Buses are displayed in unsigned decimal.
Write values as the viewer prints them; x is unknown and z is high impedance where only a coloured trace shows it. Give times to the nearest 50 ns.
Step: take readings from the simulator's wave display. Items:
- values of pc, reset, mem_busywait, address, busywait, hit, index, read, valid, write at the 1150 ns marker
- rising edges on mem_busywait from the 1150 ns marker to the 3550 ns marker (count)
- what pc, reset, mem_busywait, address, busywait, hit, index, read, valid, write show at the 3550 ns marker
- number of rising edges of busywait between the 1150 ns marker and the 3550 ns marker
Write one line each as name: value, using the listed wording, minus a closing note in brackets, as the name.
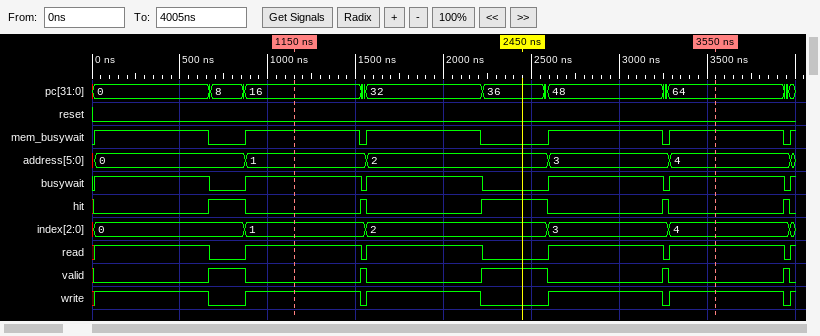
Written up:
values of pc, reset, mem_busywait, address, busywait, hit, index, read, valid, write at the 1150 ns marker: pc=16, reset=0, mem_busywait=1, address=1, busywait=1, hit=0, index=1, read=1, valid=0, write=1
rising edges on mem_busywait from the 1150 ns marker to the 3550 ns marker: 3
what pc, reset, mem_busywait, address, busywait, hit, index, read, valid, write show at the 3550 ns marker: pc=64, reset=0, mem_busywait=1, address=4, busywait=1, hit=0, index=4, read=1, valid=0, write=1
number of rising edges of busywait between the 1150 ns marker and the 3550 ns marker: 3
